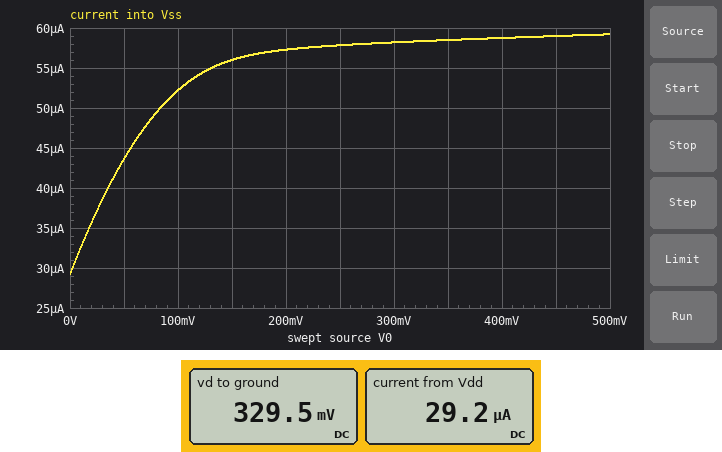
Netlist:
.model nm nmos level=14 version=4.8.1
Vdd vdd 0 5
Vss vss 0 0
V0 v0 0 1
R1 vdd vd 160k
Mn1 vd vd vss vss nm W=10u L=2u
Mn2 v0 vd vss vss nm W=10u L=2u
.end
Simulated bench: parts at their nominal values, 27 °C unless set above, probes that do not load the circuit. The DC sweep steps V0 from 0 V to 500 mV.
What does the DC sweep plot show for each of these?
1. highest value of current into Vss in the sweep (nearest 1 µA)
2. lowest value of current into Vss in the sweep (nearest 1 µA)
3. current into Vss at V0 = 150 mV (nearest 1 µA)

59 µA
29 µA
56 µA
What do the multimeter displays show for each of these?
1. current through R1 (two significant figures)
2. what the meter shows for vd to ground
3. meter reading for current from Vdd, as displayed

29 µA
329.5 mV
29.2 µA
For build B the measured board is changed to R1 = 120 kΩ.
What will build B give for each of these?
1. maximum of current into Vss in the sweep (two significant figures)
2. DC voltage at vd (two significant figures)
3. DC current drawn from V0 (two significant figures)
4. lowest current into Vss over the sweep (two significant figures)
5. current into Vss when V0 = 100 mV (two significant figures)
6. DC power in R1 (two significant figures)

78 µA
350 mV
42 µA
39 µA
68 µA
180 µW
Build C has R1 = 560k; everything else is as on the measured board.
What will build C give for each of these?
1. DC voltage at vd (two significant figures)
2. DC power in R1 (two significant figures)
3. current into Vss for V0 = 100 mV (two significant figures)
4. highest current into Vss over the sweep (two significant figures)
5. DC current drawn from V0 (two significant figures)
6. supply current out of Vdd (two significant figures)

260 mV
40 µW
16 µA
17 µA
9.7 µA
8.5 µA
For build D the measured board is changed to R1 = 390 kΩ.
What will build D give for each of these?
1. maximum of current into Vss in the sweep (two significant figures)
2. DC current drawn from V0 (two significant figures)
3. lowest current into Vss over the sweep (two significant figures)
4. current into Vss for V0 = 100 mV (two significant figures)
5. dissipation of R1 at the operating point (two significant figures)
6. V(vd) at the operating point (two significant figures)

25 µA
14 µA
12 µA
23 µA
57 µW
280 mV
